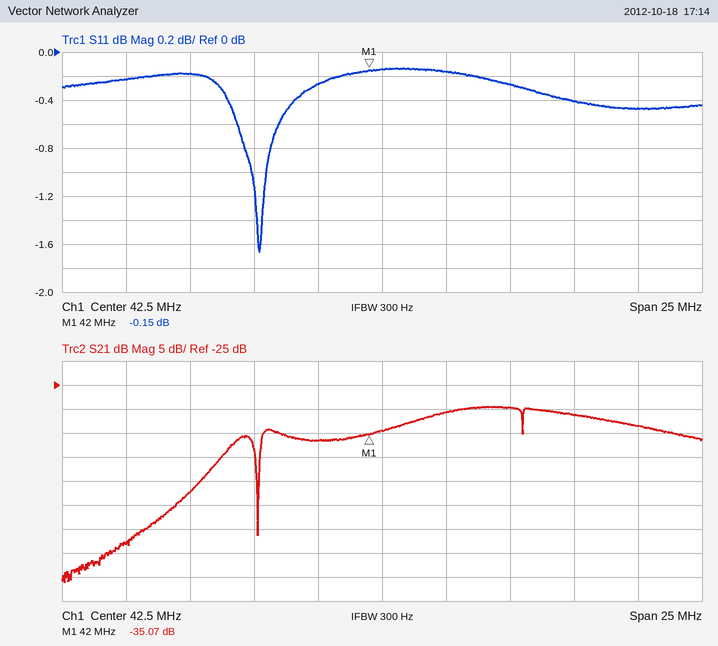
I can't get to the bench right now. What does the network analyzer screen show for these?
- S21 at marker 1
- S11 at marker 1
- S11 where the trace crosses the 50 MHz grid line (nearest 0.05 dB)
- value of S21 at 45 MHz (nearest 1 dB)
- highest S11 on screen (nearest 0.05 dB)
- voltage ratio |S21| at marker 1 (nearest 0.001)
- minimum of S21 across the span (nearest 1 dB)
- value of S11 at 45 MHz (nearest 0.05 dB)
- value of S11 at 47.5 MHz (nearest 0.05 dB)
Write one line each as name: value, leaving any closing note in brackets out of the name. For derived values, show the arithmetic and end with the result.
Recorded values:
S21 at marker 1: -35.07 dB
S11 at marker 1: -0.15 dB
S11 where the trace crosses the 50 MHz grid line: -0.40 dB
value of S21 at 45 MHz: -31 dB
highest S11 on screen: -0.15 dB
voltage ratio |S21| at marker 1: 10^(-35.07/20) ≈ 0.018
minimum of S21 across the span: -66 dB
value of S11 at 45 MHz: -0.15 dB
value of S11 at 47.5 MHz: -0.25 dB
